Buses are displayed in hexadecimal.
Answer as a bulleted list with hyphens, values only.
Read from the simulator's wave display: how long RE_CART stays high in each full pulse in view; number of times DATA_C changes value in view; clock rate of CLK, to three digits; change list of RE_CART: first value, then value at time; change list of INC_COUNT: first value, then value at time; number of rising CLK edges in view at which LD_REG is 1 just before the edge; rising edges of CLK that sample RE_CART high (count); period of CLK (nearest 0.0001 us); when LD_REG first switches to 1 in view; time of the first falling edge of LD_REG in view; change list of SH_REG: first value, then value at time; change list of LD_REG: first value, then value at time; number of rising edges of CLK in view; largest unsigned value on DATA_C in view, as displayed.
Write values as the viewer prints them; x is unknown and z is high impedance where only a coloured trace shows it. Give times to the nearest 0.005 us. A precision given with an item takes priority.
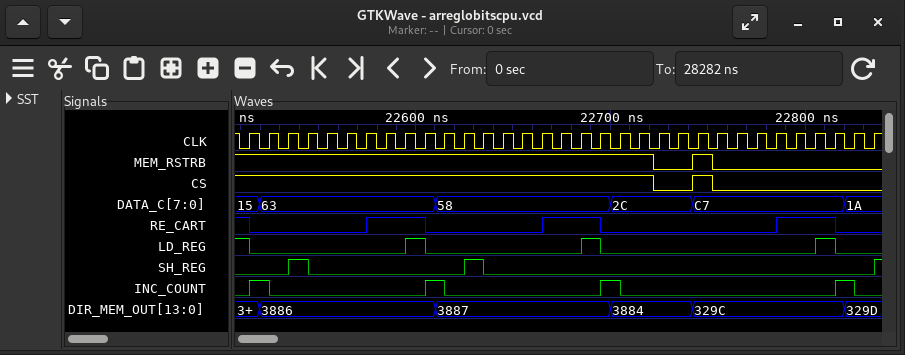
- 0.03 us, 0.03 us, 0.03 us
- 5
- 100 MHz
- 1, 0 at 22.515 us, 1 at 22.575 us, 0 at 22.605 us, 1 at 22.665 us, 0 at 22.695 us, 1 at 22.785 us, 0 at 22.815 us
- 0, 1 at 22.515 us, 0 at 22.525 us, 1 at 22.605 us, 0 at 22.615 us, 1 at 22.695 us, 0 at 22.705 us, 1 at 22.815 us, 0 at 22.825 us
- 4
- 10
- 0.01 us
- 22.595 us
- 22.515 us
- 0, 1 at 22.535 us, 0 at 22.545 us, 1 at 22.625 us, 0 at 22.635 us, 1 at 22.835 us
- 1, 0 at 22.515 us, 1 at 22.595 us, 0 at 22.605 us, 1 at 22.685 us, 0 at 22.695 us, 1 at 22.805 us, 0 at 22.815 us
- 33
- C7
